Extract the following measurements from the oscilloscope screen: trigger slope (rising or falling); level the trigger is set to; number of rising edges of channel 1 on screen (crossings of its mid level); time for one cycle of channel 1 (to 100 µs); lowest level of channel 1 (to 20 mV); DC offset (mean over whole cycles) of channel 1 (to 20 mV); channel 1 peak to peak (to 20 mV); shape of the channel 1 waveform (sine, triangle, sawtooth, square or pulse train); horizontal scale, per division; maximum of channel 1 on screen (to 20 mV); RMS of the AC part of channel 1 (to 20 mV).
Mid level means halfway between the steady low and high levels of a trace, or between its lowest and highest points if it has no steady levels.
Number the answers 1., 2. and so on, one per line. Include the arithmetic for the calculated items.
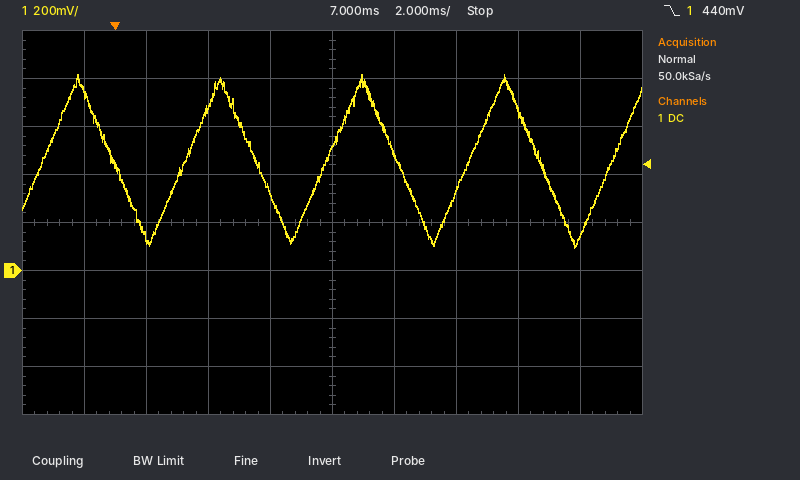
1. falling
2. 440 mV
3. 5
4. 4.6 ms
5. 100 mV
6. (820 mV + (100 mV)) / 2 ≈ 460 mV
7. 820 mV − (100 mV) = 720 mV
8. triangle
9. 2 ms
10. 820 mV
11. 720 mV / (2√3) ≈ 208 mV, so 200 mV to the nearest 20 mV
